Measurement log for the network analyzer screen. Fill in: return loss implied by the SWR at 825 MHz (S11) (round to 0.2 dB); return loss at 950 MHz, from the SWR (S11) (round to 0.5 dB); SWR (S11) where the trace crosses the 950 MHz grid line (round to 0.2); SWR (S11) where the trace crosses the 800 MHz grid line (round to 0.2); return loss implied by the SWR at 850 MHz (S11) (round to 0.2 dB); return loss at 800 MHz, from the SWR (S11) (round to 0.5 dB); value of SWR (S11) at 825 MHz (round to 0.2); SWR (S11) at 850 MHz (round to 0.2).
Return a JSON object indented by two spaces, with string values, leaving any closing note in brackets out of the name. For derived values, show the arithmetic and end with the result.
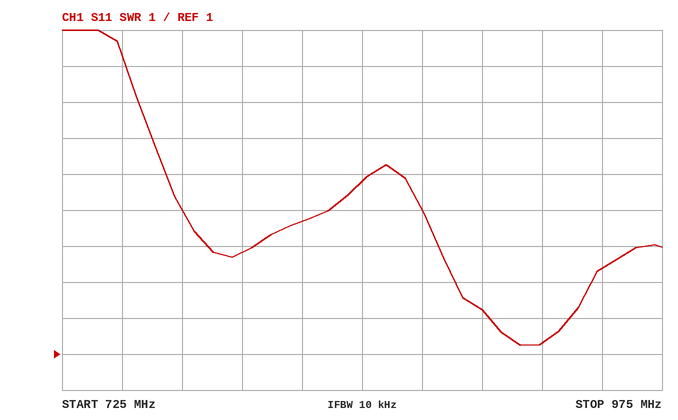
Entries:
{
  "return loss implied by the SWR at 825 MHz (S11)": "−20 log10((4.6 − 1)/(4.6 + 1)) ≈ 3.8 dB",
  "return loss at 950 MHz, from the SWR (S11)": "−20 log10((3.4 − 1)/(3.4 + 1)) ≈ 5.26 dB, so 5.5 dB to the nearest 0.5 dB",
  "SWR (S11) where the trace crosses the 950 MHz grid line": "3.4",
  "SWR (S11) where the trace crosses the 800 MHz grid line": "3.8",
  "return loss implied by the SWR at 850 MHz (S11)": "−20 log10((5.8 − 1)/(5.8 + 1)) ≈ 3.0 dB",
  "return loss at 800 MHz, from the SWR (S11)": "−20 log10((3.8 − 1)/(3.8 + 1)) ≈ 4.68 dB, so 4.5 dB to the nearest 0.5 dB",
  "value of SWR (S11) at 825 MHz": "4.6",
  "SWR (S11) at 850 MHz": "5.8"
}
